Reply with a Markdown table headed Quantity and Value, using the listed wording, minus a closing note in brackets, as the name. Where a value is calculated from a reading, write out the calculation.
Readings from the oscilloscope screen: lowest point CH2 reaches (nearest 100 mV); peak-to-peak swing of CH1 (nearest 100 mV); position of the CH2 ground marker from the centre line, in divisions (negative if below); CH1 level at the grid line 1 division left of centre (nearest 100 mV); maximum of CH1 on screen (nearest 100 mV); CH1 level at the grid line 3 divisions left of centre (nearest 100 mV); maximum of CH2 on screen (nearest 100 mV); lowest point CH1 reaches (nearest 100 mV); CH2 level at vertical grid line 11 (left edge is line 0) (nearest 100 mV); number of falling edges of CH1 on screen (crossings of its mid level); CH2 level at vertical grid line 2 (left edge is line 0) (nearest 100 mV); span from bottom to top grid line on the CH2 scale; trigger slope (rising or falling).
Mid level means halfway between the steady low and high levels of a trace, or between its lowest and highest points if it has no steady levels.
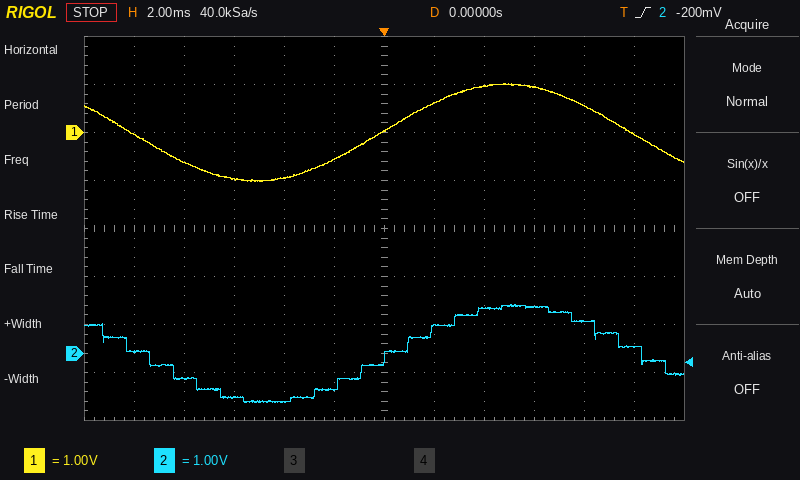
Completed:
| Quantity | Value |
|---|---|
| lowest point CH2 reaches | -1.0 V |
| peak-to-peak swing of CH1 | 1.0 V − (-1.0 V) = 2.0 V |
| position of the CH2 ground marker from the centre line, in divisions | -2.6 div |
| CH1 level at the grid line 1 division left of centre | -600 mV |
| maximum of CH1 on screen | 1.0 V |
| CH1 level at the grid line 3 divisions left of centre | -1.0 V |
| maximum of CH2 on screen | 1.0 V |
| lowest point CH1 reaches | -1.0 V |
| CH2 level at vertical grid line 11 (left edge is line 0) | 100 mV |
| number of falling edges of CH1 on screen | 2 |
| CH2 level at vertical grid line 2 (left edge is line 0) | -500 mV |
| span from bottom to top grid line on the CH2 scale | 8 V |
| trigger slope | rising |
